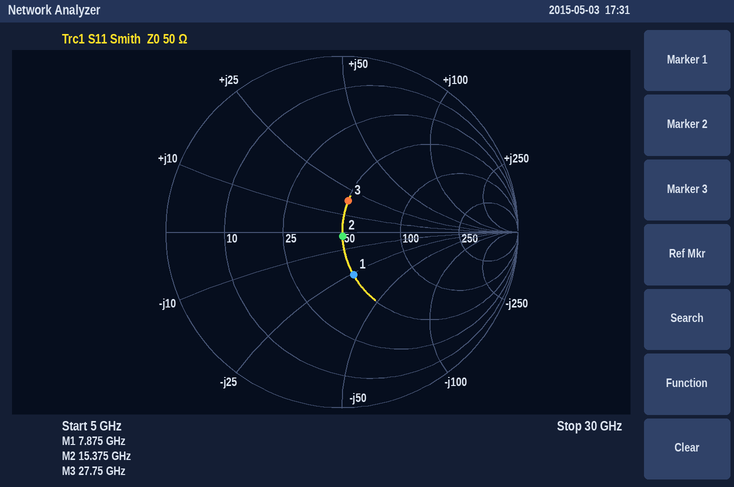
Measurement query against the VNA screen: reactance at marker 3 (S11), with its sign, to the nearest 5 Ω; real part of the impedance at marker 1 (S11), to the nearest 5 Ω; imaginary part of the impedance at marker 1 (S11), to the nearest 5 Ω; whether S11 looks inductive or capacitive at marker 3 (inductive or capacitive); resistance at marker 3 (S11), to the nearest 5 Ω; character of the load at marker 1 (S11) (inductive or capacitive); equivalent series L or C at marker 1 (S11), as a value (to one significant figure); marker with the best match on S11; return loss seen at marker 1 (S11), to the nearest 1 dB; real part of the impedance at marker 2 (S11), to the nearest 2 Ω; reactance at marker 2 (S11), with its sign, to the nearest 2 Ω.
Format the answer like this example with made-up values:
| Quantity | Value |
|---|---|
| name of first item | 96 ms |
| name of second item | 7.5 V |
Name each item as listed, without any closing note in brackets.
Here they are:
| Quantity | Value |
|---|---|
| reactance at marker 3 (S11), with its sign, to the nearest 5 Ω | +20 Ω |
| real part of the impedance at marker 1 (S11), to the nearest 5 Ω | 50 Ω |
| imaginary part of the impedance at marker 1 (S11), to the nearest 5 Ω | -25 Ω |
| whether S11 looks inductive or capacitive at marker 3 | inductive |
| resistance at marker 3 (S11), to the nearest 5 Ω | 50 Ω |
| character of the load at marker 1 (S11) | capacitive |
| equivalent series L or C at marker 1 (S11), as a value | 800 fF |
| marker with the best match on S11 | marker 2 |
| return loss seen at marker 1 (S11), to the nearest 1 dB | 12 dB |
| real part of the impedance at marker 2 (S11), to the nearest 2 Ω | 50 Ω |
| reactance at marker 2 (S11), with its sign, to the nearest 2 Ω | -2 Ω |
